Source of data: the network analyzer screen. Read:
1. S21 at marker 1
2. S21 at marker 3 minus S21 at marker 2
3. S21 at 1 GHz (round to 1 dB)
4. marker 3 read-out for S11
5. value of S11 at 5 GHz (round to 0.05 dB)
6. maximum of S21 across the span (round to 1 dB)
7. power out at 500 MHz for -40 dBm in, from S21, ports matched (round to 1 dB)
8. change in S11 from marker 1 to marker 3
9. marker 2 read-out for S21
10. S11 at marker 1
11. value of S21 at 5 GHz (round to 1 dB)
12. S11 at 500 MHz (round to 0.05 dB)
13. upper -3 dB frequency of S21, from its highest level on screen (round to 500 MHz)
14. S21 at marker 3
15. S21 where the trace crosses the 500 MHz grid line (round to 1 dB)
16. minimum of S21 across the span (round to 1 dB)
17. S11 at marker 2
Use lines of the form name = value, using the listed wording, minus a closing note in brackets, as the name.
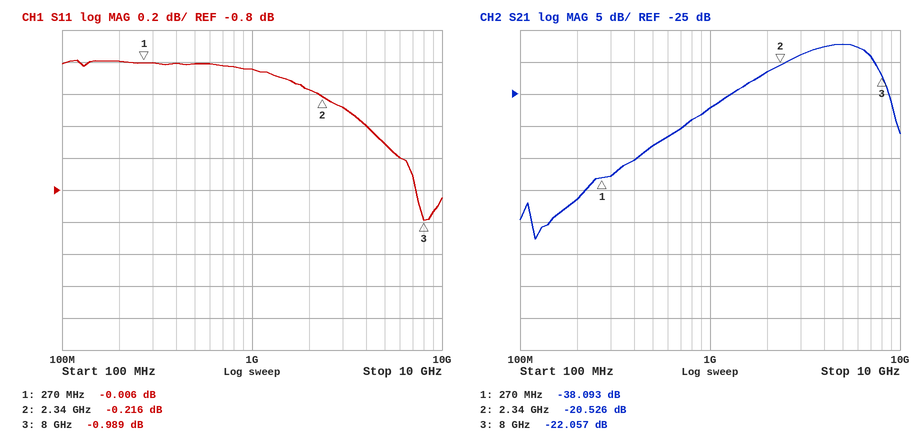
S21 at marker 1 = -38.093 dB
S21 at marker 3 minus S21 at marker 2 = -1.531 dB
S21 at 1 GHz = -27 dB
marker 3 read-out for S11 = -0.989 dB
value of S11 at 5 GHz = -0.50 dB
maximum of S21 across the span = -17 dB
power out at 500 MHz for -40 dBm in, from S21, ports matched = -73 dBm
change in S11 from marker 1 to marker 3 = -0.983 dB
marker 2 read-out for S21 = -20.526 dB
S11 at marker 1 = -0.006 dB
value of S21 at 5 GHz = -17 dB
S11 at 500 MHz = 0.00 dB
upper -3 dB frequency of S21, from its highest level on screen = 7.5 GHz
S21 at marker 3 = -22.057 dB
S21 where the trace crosses the 500 MHz grid line = -33 dB
minimum of S21 across the span = -48 dB
S11 at marker 2 = -0.216 dB
